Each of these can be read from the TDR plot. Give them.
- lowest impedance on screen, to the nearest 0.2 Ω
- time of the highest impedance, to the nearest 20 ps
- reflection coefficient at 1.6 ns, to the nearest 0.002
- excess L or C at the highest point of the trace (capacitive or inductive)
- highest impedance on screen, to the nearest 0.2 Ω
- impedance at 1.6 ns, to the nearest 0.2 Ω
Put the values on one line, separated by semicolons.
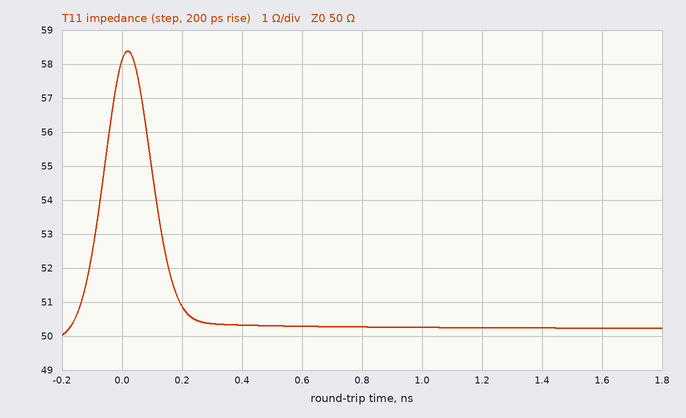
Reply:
50.0 Ω; 20 ps; +0.002; inductive; 58.4 Ω; 50.2 Ω
